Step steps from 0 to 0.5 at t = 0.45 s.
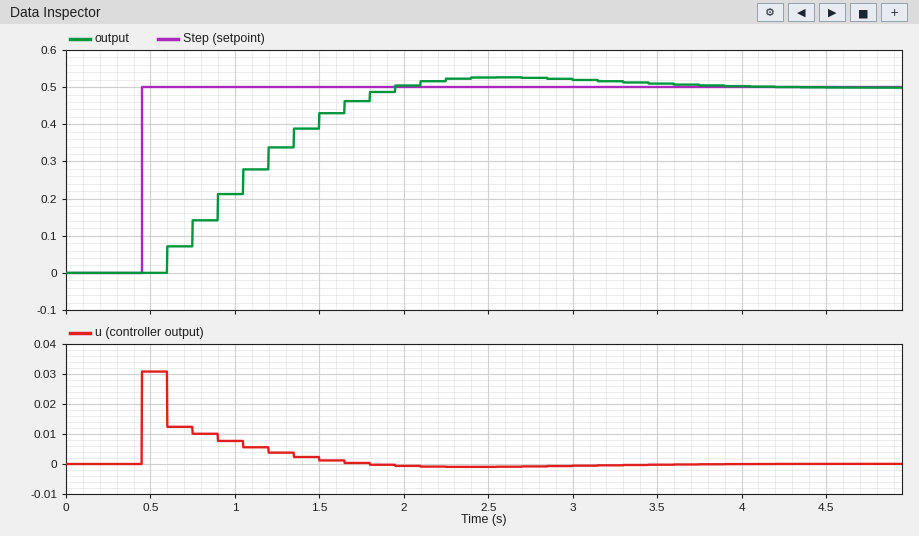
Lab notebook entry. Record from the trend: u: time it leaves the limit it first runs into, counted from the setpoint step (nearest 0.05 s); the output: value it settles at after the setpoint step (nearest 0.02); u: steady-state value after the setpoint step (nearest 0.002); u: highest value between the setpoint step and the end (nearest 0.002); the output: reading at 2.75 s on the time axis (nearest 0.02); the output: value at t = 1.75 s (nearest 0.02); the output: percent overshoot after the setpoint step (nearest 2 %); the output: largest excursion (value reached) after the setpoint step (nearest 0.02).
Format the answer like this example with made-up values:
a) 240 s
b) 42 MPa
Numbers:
a) 0.15 s
b) 0.50
c) 0.000
d) 0.030
e) 0.52
f) 0.46
g) 6 %
h) 0.52
